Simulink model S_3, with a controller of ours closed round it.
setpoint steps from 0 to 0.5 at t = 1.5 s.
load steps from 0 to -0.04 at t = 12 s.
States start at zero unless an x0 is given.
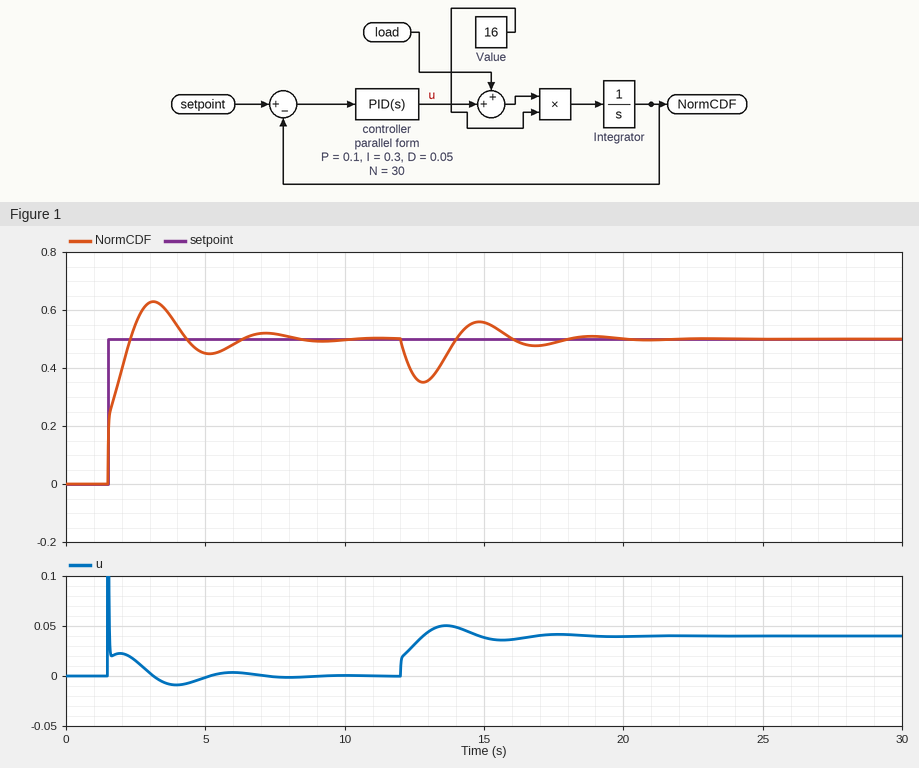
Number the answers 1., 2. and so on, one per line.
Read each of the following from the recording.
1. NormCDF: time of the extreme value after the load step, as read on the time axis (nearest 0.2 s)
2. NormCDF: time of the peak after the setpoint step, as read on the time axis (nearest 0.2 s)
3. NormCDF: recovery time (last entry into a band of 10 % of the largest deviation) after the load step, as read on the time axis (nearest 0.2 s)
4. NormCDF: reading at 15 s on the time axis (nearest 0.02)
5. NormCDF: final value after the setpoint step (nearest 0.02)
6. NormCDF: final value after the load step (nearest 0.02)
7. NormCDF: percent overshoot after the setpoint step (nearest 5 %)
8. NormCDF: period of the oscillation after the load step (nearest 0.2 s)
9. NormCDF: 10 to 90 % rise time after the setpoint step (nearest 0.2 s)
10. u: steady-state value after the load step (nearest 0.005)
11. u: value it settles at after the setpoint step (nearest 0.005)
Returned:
1. 12.8 s
2. 3.2 s
3. 17.4 s
4. 0.56
5. 0.50
6. 0.50
7. 25 %
8. 4.0 s
9. 0.6 s
10. 0.040
11. 0.000
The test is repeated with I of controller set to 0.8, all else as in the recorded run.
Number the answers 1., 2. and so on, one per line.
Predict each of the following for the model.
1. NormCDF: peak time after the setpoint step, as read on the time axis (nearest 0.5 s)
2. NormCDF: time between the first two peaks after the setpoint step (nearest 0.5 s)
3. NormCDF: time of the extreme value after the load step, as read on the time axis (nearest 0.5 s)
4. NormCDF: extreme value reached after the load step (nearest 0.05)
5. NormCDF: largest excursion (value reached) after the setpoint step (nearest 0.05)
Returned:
1. 2.5 s
2. 2.5 s
3. 12.5 s
4. 0.40
5. 0.65
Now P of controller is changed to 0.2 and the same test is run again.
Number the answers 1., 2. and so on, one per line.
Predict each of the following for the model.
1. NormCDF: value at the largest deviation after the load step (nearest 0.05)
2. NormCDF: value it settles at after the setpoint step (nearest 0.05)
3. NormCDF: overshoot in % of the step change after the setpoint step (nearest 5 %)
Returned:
1. 0.40
2. 0.50
3. 15 %
